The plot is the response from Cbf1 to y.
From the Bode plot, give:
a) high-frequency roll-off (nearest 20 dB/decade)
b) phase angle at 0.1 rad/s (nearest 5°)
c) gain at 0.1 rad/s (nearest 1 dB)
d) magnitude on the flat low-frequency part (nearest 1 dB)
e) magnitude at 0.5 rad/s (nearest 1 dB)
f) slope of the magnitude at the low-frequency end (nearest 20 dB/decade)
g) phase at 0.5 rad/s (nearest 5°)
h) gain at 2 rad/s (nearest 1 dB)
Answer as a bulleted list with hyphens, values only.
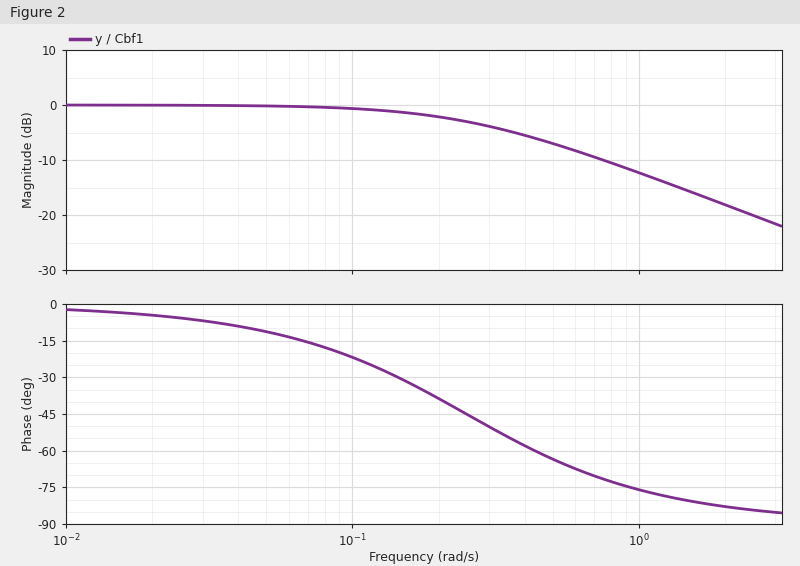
- -20 dB/decade
- -20°
- -1 dB
- 0 dB
- -7 dB
- 0 dB/decade
- -65°
- -18 dB
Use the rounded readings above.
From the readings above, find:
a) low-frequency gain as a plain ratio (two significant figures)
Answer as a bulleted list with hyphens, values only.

- 1.0
